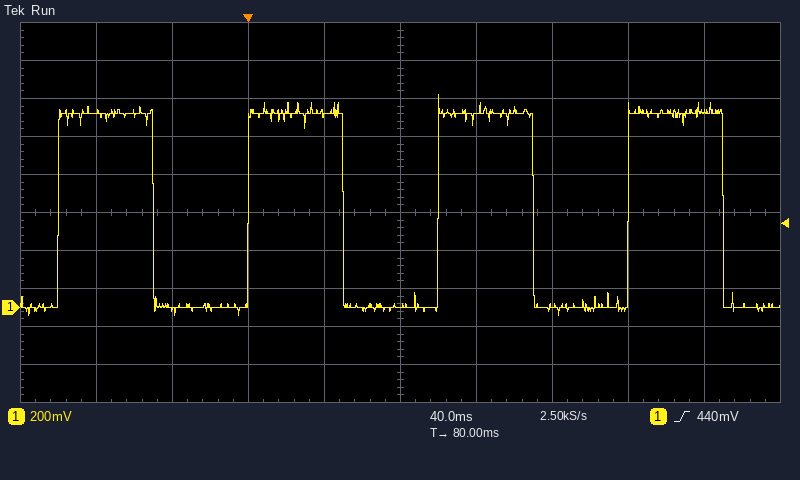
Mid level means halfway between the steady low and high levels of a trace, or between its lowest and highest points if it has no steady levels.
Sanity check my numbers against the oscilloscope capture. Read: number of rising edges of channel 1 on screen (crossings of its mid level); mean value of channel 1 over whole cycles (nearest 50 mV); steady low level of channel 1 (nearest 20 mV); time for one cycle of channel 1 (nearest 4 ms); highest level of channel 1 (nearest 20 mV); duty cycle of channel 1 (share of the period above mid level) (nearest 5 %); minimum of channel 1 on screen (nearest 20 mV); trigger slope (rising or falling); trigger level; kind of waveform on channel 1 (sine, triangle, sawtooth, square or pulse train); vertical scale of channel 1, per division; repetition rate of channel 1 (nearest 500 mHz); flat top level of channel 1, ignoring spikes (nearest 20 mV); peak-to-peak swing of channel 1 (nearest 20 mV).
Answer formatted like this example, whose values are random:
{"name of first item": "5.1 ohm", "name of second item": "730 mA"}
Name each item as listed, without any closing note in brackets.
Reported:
{"number of rising edges of channel 1 on screen": "4", "mean value of channel 1 over whole cycles": "500 mV", "steady low level of channel 1": "0 mV", "time for one cycle of channel 1": "100 ms", "highest level of channel 1": "1.12 V", "duty cycle of channel 1 (share of the period above mid level)": "50 %", "minimum of channel 1 on screen": "-40 mV", "trigger slope": "rising", "trigger level": "440 mV", "kind of waveform on channel 1": "square", "vertical scale of channel 1, per division": "200 mV", "repetition rate of channel 1": "10.0 Hz", "flat top level of channel 1, ignoring spikes": "1.02 V", "peak-to-peak swing of channel 1": "1.16 V"}
